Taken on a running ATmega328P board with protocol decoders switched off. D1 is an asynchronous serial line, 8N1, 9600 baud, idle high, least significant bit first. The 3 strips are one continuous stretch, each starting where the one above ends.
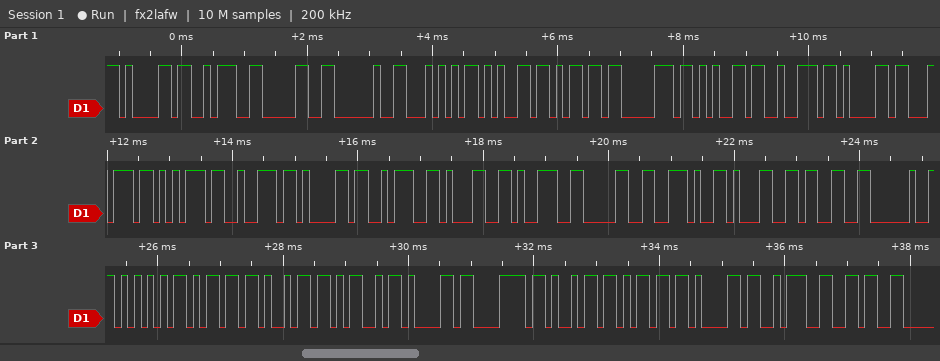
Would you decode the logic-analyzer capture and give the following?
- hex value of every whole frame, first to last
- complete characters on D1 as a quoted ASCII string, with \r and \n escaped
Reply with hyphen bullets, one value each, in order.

- 61 3A 30 20 54 65 6D 70 65 72 61 74 75 72 61 3A 31 39 30 2E 31 33 20 55 6D 69 4D 61 78 69 6D 61 3A 36
- "a:0 Temperatura:190.13 UmiMaxima:6"
